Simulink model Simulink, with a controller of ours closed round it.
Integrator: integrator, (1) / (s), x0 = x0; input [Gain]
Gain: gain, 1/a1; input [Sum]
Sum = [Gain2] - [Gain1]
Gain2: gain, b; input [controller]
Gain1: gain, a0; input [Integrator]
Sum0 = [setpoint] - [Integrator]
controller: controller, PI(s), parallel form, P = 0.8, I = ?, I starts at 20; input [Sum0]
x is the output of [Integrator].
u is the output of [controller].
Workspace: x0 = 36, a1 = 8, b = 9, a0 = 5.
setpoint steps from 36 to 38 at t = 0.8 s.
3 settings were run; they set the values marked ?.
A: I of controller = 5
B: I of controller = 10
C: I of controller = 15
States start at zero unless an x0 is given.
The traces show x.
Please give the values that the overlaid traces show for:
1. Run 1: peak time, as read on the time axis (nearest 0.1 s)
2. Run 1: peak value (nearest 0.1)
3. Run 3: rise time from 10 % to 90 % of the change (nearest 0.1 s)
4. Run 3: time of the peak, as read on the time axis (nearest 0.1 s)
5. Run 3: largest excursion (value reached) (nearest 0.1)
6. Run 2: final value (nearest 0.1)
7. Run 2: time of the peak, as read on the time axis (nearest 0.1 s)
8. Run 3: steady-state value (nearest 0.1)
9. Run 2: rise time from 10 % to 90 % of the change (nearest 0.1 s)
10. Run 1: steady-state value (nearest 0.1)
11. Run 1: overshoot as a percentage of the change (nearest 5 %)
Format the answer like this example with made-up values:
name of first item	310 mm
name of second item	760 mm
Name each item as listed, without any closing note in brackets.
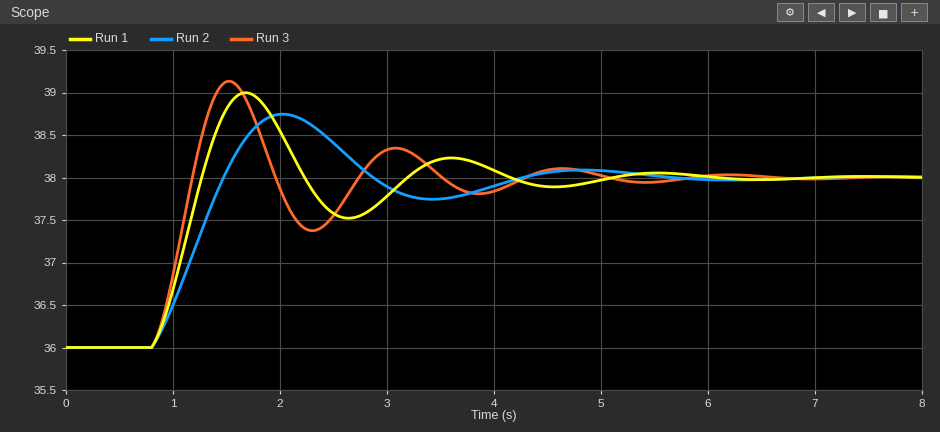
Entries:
Run 1: peak time, as read on the time axis	1.7 s
Run 1: peak value	39.0
Run 3: rise time from 10 % to 90 % of the change	0.3 s
Run 3: time of the peak, as read on the time axis	1.5 s
Run 3: largest excursion (value reached)	39.1
Run 2: final value	38.0
Run 2: time of the peak, as read on the time axis	2.0 s
Run 3: steady-state value	38.0
Run 2: rise time from 10 % to 90 % of the change	0.5 s
Run 1: steady-state value	38.0
Run 1: overshoot as a percentage of the change	50 %
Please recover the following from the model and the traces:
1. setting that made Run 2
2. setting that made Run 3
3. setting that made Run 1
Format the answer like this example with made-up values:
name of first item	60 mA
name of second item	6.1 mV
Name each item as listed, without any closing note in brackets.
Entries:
setting that made Run 2	A
setting that made Run 3	C
setting that made Run 1	B
